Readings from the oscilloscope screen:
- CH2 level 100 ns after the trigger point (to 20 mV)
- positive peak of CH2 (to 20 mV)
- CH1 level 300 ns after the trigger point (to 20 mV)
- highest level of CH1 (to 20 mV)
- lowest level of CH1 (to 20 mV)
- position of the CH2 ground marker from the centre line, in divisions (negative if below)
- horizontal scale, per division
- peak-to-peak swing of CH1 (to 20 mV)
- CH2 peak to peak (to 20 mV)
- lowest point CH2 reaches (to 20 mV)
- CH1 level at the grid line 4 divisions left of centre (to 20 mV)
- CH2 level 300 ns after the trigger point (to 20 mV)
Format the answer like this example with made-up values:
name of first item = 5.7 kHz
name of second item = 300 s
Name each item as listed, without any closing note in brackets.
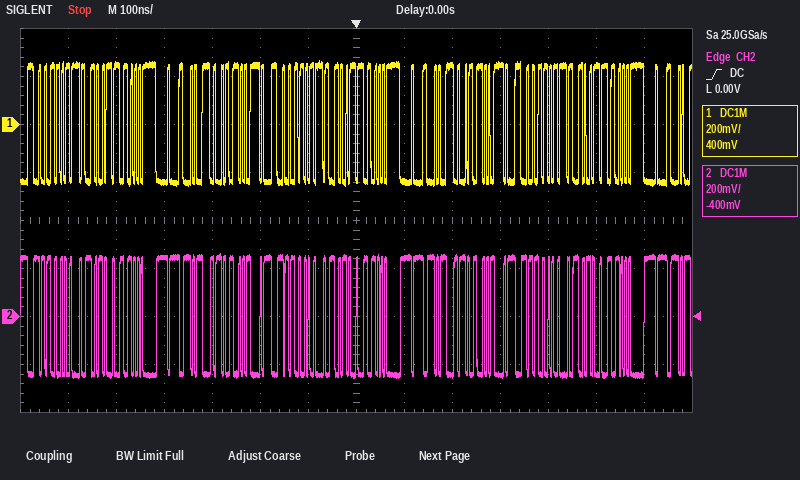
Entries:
CH2 level 100 ns after the trigger point = 240 mV
positive peak of CH2 = 260 mV
CH1 level 300 ns after the trigger point = 240 mV
highest level of CH1 = 260 mV
lowest level of CH1 = -260 mV
position of the CH2 ground marker from the centre line, in divisions = -2.0 div
horizontal scale, per division = 100 ns
peak-to-peak swing of CH1 = 520 mV
CH2 peak to peak = 520 mV
lowest point CH2 reaches = -260 mV
CH1 level at the grid line 4 divisions left of centre = -240 mV
CH2 level 300 ns after the trigger point = -240 mV
